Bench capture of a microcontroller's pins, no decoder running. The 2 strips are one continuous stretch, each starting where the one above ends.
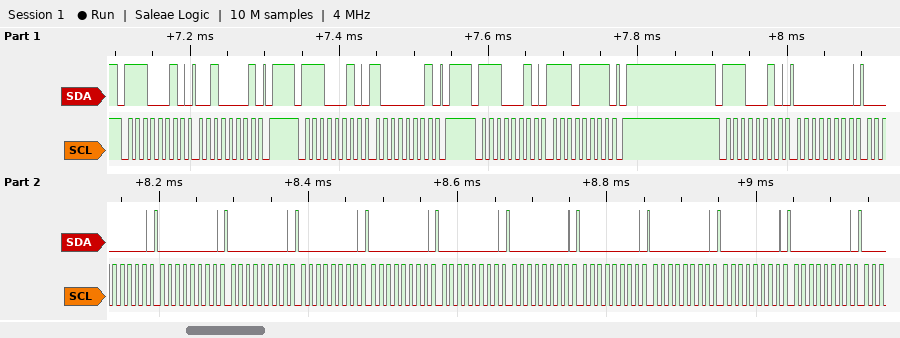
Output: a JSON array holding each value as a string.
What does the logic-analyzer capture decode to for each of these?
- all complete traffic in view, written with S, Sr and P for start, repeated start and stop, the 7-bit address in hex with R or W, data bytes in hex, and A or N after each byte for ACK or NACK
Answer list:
["S 71W A 21 A P S 71W A 81 A P S 71W A EF A P S 71W A 00 A 00 A 00 A 00 A 00 A 00 A 00 A 00 A 00 A 00 A 00 A 00 A"]
